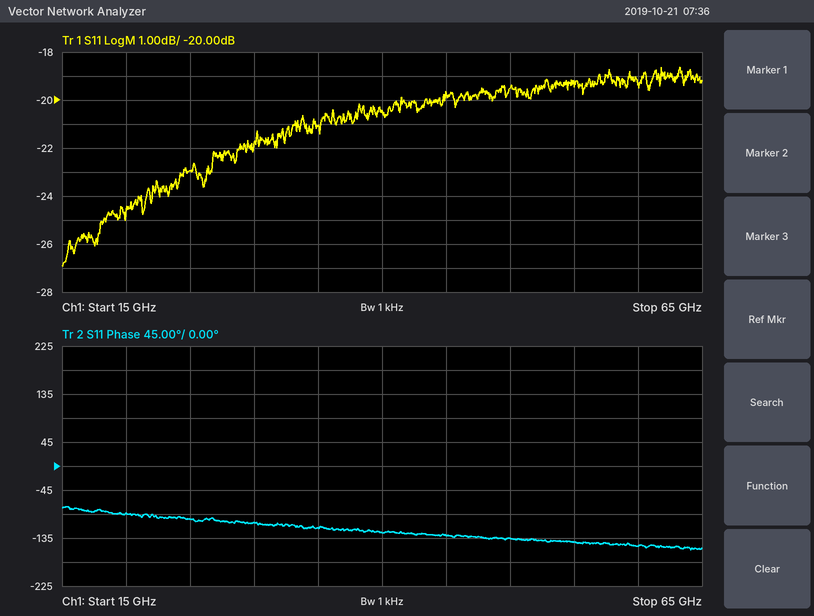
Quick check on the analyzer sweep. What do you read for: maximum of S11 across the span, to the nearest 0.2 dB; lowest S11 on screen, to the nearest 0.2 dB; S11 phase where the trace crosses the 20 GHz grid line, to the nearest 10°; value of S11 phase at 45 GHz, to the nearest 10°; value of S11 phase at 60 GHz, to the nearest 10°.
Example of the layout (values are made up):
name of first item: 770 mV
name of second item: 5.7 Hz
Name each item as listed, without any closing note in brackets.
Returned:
maximum of S11 across the span, to the nearest 0.2 dB: -18.6 dB
lowest S11 on screen, to the nearest 0.2 dB: -27.0 dB
S11 phase where the trace crosses the 20 GHz grid line, to the nearest 10°: -90°
value of S11 phase at 45 GHz, to the nearest 10°: -130°
value of S11 phase at 60 GHz, to the nearest 10°: -150°
